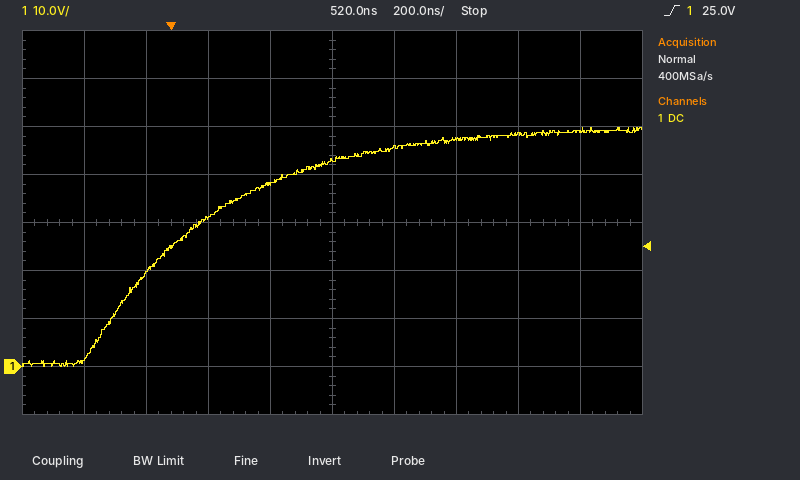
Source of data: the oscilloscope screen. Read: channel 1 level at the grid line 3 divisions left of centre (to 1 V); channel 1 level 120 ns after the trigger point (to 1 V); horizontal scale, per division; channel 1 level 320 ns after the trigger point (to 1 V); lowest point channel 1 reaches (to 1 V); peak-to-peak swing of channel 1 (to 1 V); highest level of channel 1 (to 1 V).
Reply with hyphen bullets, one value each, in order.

- 20 V
- 31 V
- 200 ns
- 38 V
- 0 V
- 50 V
- 50 V
